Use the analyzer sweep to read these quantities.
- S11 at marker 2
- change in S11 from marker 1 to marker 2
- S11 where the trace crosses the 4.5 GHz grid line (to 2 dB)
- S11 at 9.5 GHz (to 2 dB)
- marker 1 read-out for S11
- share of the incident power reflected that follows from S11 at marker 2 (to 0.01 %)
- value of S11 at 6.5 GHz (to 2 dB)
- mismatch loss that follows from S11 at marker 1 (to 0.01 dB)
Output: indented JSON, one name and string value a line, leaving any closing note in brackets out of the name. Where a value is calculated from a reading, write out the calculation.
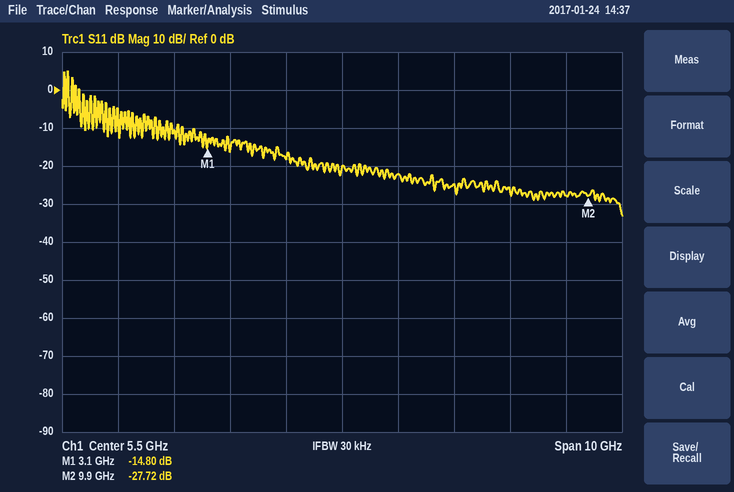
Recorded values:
{
  "S11 at marker 2": "-27.72 dB",
  "change in S11 from marker 1 to marker 2": "-27.72 − (-14.8) = -12.92 dB",
  "S11 where the trace crosses the 4.5 GHz grid line": "-18 dB",
  "S11 at 9.5 GHz": "-28 dB",
  "marker 1 read-out for S11": "-14.80 dB",
  "share of the incident power reflected that follows from S11 at marker 2": "10^(-27.72/10) ≈ 0.17 %",
  "value of S11 at 6.5 GHz": "-22 dB",
  "mismatch loss that follows from S11 at marker 1": "−10 log10(1 − 10^(-14.8/10)) ≈ 0.15 dB"
}
